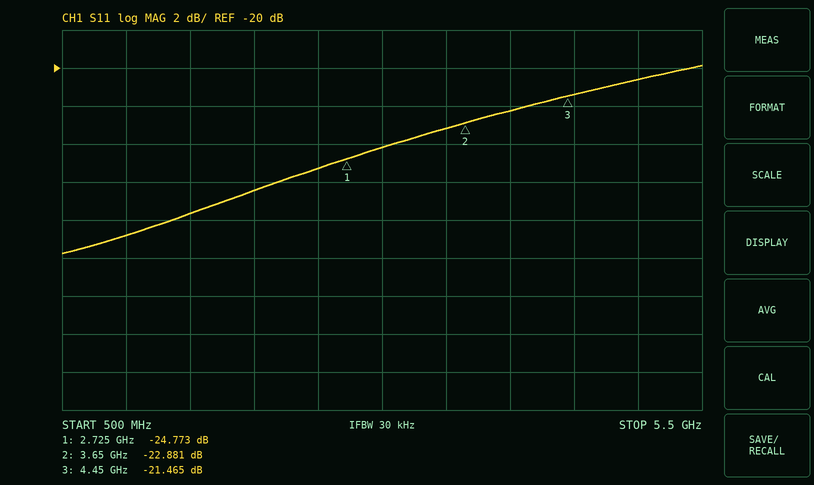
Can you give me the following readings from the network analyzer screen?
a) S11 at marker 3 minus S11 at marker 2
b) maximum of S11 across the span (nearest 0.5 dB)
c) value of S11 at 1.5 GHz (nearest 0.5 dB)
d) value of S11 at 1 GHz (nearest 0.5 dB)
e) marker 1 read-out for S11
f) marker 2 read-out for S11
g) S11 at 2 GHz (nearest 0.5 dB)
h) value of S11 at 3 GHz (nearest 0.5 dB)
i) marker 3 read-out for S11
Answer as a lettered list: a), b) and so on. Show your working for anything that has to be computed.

a) -21.465 − (-22.881) = 1.416 dB
b) -20.0 dB
c) -27.5 dB
d) -29.0 dB
e) -24.773 dB
f) -22.881 dB
g) -26.5 dB
h) -24.0 dB
i) -21.465 dB
